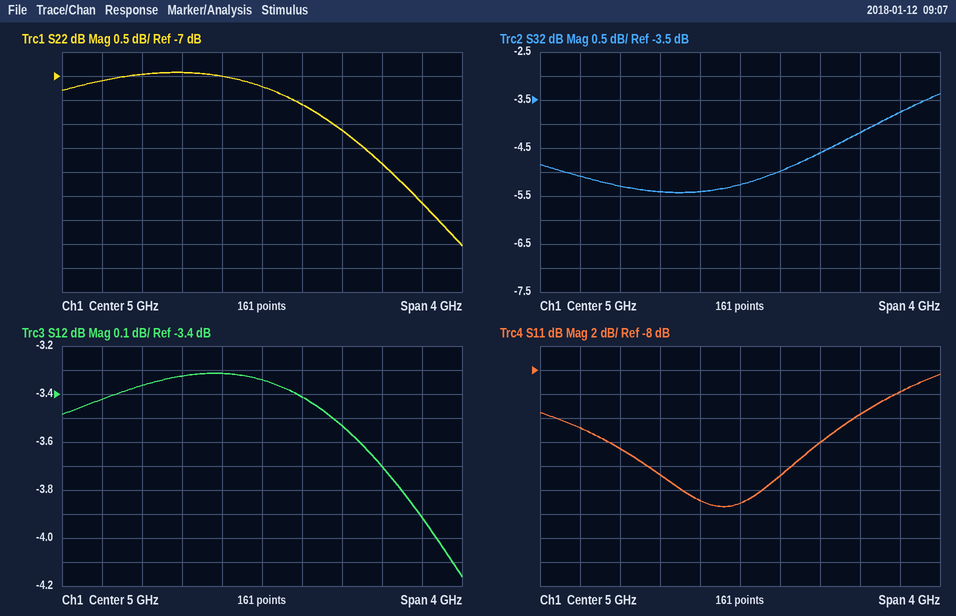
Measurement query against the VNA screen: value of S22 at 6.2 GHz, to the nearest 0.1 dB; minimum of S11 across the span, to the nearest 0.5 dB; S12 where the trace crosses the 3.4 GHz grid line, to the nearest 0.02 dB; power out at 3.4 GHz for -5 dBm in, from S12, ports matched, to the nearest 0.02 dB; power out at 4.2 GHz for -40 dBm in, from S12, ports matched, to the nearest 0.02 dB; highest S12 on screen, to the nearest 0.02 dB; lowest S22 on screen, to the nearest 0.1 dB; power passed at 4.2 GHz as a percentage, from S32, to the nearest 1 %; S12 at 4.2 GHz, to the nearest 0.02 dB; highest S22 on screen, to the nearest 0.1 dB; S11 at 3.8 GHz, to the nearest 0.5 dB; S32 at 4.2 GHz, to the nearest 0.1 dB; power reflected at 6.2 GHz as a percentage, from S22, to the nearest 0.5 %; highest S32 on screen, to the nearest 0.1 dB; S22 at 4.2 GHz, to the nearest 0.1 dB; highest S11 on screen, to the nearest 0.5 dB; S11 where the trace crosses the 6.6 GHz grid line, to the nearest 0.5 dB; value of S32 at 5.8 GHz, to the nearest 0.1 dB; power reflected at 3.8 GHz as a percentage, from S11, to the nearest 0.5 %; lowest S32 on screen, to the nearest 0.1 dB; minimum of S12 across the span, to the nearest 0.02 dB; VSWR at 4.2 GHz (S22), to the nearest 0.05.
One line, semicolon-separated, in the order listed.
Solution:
-8.8 dB; -19.5 dB; -3.42 dB; -8.42 dBm; -43.32 dBm; -3.32 dB; -10.5 dB; 29 %; -3.32 dB; -6.9 dB; -14.5 dB; -5.4 dB; 13.0 %; -3.4 dB; -6.9 dB; -8.5 dB; -10.0 dB; -4.6 dB; 3.5 %; -5.4 dB; -4.16 dB; 2.65
